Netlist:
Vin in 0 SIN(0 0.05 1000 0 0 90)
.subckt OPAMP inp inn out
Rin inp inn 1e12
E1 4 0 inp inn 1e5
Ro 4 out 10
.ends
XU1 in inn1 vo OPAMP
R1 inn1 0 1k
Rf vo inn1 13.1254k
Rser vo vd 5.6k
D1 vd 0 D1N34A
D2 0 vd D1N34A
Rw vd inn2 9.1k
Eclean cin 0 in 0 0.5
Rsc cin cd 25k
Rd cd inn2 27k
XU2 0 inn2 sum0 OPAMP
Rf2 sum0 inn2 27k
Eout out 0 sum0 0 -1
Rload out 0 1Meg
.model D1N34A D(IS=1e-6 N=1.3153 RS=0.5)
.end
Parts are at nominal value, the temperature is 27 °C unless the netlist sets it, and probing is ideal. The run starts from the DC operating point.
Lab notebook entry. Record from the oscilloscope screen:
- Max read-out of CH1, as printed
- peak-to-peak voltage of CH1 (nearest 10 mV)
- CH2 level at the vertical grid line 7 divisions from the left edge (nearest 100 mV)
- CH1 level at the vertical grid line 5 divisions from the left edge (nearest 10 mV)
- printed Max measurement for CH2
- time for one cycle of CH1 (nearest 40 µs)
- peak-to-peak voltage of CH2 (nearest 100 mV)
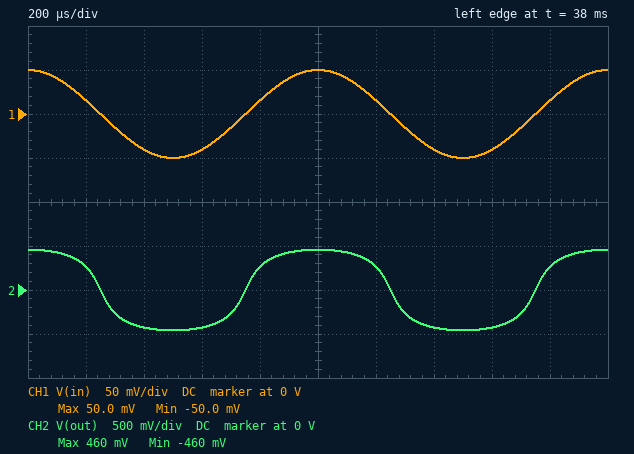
50.0 mV
100 mV
-400 mV
50 mV
460 mV
1.00 ms
900 mV
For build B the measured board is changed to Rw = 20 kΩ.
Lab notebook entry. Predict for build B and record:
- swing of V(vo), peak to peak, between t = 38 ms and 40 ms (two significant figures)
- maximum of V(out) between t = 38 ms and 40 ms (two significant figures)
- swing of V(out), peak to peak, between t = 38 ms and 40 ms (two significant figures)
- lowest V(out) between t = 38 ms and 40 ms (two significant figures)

1.4 V
220 mV
440 mV
-220 mV
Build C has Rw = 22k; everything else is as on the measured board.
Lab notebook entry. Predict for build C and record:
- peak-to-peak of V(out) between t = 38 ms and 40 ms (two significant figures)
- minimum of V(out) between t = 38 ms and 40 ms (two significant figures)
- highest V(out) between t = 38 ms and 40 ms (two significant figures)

400 mV
-200 mV
200 mV
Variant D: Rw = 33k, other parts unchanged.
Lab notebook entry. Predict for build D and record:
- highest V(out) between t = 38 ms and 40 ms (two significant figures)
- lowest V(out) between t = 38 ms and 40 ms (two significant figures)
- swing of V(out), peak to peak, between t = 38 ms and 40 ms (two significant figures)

140 mV
-140 mV
280 mV
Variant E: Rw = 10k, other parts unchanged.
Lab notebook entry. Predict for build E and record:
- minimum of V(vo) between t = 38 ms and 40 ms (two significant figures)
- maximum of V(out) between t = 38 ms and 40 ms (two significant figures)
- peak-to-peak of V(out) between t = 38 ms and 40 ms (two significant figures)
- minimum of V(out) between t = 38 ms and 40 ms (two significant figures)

-710 mV
420 mV
840 mV
-420 mV
